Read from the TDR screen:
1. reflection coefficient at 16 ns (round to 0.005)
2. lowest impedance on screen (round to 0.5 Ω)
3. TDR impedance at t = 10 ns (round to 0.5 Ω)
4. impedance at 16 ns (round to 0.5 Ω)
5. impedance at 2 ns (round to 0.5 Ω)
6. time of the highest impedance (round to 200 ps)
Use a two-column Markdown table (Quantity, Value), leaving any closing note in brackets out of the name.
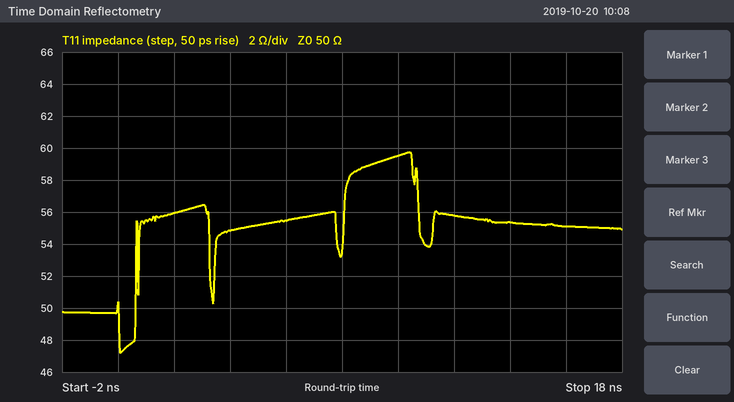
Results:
| Quantity | Value |
|---|---|
| reflection coefficient at 16 ns | +0.050 |
| lowest impedance on screen | 47.0 Ω |
| TDR impedance at t = 10 ns | 59.5 Ω |
| impedance at 16 ns | 55.0 Ω |
| impedance at 2 ns | 56.0 Ω |
| time of the highest impedance | 10.4 ns |
